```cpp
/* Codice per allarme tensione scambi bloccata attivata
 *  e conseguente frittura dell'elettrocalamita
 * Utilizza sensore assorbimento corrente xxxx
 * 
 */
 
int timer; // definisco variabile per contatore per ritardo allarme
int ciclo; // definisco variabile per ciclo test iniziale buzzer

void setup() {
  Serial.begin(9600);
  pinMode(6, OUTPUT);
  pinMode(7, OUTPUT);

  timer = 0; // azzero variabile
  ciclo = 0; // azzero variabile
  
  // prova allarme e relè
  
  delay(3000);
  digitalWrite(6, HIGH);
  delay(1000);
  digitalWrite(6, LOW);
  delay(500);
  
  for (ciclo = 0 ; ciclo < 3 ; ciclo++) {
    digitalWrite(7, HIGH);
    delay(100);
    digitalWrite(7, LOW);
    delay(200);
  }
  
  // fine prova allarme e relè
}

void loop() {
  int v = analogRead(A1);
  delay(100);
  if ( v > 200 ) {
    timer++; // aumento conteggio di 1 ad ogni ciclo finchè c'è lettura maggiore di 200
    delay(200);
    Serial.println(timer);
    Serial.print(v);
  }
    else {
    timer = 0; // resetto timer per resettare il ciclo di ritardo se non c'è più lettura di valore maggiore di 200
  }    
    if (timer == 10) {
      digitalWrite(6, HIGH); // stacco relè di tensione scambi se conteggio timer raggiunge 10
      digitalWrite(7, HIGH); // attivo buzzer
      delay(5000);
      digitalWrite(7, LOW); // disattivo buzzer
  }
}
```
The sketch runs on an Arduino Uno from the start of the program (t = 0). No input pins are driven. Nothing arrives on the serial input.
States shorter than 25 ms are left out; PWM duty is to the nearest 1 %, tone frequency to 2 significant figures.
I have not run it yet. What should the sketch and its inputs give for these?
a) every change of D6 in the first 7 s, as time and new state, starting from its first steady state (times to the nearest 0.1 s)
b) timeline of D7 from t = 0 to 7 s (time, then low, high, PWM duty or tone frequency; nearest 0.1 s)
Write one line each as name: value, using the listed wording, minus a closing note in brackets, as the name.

every change of D6 in the first 7 s, as time and new state, starting from its first steady state: 0 s low; 3 s high; 4 s low
timeline of D7 from t = 0 to 7 s: 0 s low; 4.5 s high; 4.6 s low; 4.8 s high; 4.9 s low; 5.1 s high; 5.2 s low
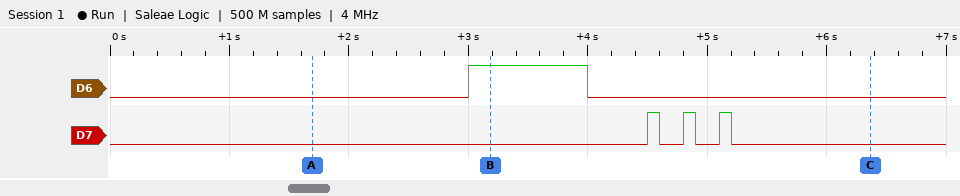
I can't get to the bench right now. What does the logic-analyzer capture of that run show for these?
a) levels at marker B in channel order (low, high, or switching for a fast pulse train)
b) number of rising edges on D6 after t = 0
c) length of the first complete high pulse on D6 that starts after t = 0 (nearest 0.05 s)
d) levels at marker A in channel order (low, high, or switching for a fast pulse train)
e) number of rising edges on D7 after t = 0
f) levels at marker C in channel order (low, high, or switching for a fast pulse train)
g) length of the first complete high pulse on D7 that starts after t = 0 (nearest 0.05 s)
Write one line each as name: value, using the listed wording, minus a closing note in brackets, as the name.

levels at marker B in channel order: D6 high, D7 low
number of rising edges on D6 after t = 0: 1
length of the first complete high pulse on D6 that starts after t = 0: 1.00 s
levels at marker A in channel order: D6 low, D7 low
number of rising edges on D7 after t = 0: 3
levels at marker C in channel order: D6 low, D7 low
length of the first complete high pulse on D7 that starts after t = 0: 0.10 s
